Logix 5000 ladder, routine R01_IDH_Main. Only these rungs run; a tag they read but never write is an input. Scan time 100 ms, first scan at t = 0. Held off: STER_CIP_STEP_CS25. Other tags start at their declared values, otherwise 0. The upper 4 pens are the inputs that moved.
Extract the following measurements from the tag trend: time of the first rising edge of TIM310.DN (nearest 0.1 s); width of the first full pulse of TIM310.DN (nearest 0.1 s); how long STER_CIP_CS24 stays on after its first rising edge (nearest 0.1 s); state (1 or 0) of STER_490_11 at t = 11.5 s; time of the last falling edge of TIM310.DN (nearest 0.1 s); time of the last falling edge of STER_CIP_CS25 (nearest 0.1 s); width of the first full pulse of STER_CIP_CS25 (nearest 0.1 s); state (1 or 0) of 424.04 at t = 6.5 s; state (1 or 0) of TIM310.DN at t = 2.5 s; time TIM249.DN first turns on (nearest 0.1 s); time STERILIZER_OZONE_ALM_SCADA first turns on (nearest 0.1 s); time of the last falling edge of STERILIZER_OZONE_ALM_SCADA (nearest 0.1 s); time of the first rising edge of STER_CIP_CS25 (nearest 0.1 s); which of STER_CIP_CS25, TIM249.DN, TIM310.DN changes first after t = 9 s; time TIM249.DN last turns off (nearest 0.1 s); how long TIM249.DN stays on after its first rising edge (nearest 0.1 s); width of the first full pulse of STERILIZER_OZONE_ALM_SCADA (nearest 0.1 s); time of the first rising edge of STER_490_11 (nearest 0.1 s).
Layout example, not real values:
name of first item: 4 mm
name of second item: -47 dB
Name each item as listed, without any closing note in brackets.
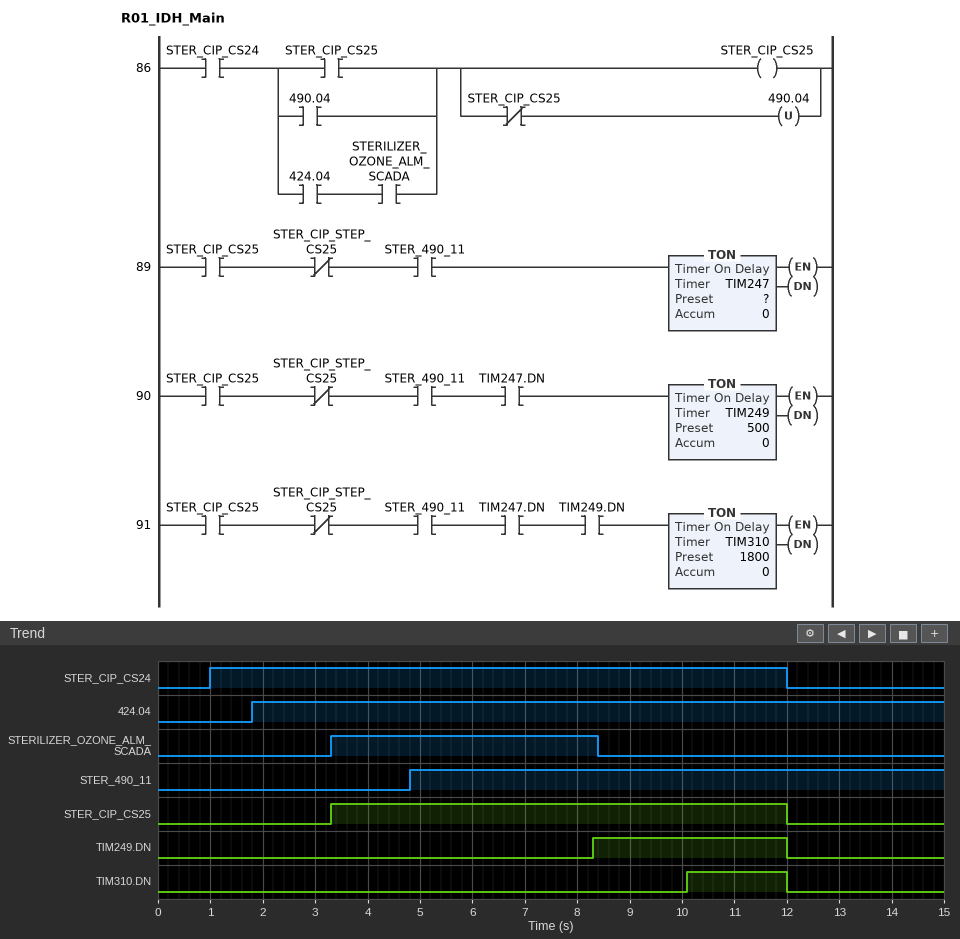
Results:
time of the first rising edge of TIM310.DN: 10.1 s
width of the first full pulse of TIM310.DN: 1.9 s
how long STER_CIP_CS24 stays on after its first rising edge: 11.0 s
state (1 or 0) of STER_490_11 at t = 11.5 s: 1
time of the last falling edge of TIM310.DN: 12.0 s
time of the last falling edge of STER_CIP_CS25: 12.0 s
width of the first full pulse of STER_CIP_CS25: 8.7 s
state (1 or 0) of 424.04 at t = 6.5 s: 1
state (1 or 0) of TIM310.DN at t = 2.5 s: 0
time TIM249.DN first turns on: 8.3 s
time STERILIZER_OZONE_ALM_SCADA first turns on: 3.3 s
time of the last falling edge of STERILIZER_OZONE_ALM_SCADA: 8.4 s
time of the first rising edge of STER_CIP_CS25: 3.3 s
which of STER_CIP_CS25, TIM249.DN, TIM310.DN changes first after t = 9 s: TIM310.DN
time TIM249.DN last turns off: 12.0 s
how long TIM249.DN stays on after its first rising edge: 3.7 s
width of the first full pulse of STERILIZER_OZONE_ALM_SCADA: 5.1 s
time of the first rising edge of STER_490_11: 4.8 s
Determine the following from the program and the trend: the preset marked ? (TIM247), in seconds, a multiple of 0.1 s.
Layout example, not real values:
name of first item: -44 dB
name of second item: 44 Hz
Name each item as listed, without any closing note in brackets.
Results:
the preset marked ? (TIM247), in seconds, a multiple of 0.1 s: 3.0 s
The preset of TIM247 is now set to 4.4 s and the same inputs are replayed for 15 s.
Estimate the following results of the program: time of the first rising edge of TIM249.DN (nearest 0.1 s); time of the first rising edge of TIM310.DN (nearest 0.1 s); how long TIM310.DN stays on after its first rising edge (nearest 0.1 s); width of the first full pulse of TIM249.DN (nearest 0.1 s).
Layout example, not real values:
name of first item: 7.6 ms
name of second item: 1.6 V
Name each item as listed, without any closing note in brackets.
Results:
time of the first rising edge of TIM249.DN: 9.7 s
time of the first rising edge of TIM310.DN: 11.5 s
how long TIM310.DN stays on after its first rising edge: 0.5 s
width of the first full pulse of TIM249.DN: 2.3 s
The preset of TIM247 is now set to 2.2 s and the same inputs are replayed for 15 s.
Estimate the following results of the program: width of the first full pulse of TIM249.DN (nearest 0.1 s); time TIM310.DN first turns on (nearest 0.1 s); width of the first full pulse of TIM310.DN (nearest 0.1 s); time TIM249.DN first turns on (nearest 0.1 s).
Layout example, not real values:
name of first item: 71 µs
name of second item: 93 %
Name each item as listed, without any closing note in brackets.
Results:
width of the first full pulse of TIM249.DN: 4.5 s
time TIM310.DN first turns on: 9.3 s
width of the first full pulse of TIM310.DN: 2.7 s
time TIM249.DN first turns on: 7.5 s
